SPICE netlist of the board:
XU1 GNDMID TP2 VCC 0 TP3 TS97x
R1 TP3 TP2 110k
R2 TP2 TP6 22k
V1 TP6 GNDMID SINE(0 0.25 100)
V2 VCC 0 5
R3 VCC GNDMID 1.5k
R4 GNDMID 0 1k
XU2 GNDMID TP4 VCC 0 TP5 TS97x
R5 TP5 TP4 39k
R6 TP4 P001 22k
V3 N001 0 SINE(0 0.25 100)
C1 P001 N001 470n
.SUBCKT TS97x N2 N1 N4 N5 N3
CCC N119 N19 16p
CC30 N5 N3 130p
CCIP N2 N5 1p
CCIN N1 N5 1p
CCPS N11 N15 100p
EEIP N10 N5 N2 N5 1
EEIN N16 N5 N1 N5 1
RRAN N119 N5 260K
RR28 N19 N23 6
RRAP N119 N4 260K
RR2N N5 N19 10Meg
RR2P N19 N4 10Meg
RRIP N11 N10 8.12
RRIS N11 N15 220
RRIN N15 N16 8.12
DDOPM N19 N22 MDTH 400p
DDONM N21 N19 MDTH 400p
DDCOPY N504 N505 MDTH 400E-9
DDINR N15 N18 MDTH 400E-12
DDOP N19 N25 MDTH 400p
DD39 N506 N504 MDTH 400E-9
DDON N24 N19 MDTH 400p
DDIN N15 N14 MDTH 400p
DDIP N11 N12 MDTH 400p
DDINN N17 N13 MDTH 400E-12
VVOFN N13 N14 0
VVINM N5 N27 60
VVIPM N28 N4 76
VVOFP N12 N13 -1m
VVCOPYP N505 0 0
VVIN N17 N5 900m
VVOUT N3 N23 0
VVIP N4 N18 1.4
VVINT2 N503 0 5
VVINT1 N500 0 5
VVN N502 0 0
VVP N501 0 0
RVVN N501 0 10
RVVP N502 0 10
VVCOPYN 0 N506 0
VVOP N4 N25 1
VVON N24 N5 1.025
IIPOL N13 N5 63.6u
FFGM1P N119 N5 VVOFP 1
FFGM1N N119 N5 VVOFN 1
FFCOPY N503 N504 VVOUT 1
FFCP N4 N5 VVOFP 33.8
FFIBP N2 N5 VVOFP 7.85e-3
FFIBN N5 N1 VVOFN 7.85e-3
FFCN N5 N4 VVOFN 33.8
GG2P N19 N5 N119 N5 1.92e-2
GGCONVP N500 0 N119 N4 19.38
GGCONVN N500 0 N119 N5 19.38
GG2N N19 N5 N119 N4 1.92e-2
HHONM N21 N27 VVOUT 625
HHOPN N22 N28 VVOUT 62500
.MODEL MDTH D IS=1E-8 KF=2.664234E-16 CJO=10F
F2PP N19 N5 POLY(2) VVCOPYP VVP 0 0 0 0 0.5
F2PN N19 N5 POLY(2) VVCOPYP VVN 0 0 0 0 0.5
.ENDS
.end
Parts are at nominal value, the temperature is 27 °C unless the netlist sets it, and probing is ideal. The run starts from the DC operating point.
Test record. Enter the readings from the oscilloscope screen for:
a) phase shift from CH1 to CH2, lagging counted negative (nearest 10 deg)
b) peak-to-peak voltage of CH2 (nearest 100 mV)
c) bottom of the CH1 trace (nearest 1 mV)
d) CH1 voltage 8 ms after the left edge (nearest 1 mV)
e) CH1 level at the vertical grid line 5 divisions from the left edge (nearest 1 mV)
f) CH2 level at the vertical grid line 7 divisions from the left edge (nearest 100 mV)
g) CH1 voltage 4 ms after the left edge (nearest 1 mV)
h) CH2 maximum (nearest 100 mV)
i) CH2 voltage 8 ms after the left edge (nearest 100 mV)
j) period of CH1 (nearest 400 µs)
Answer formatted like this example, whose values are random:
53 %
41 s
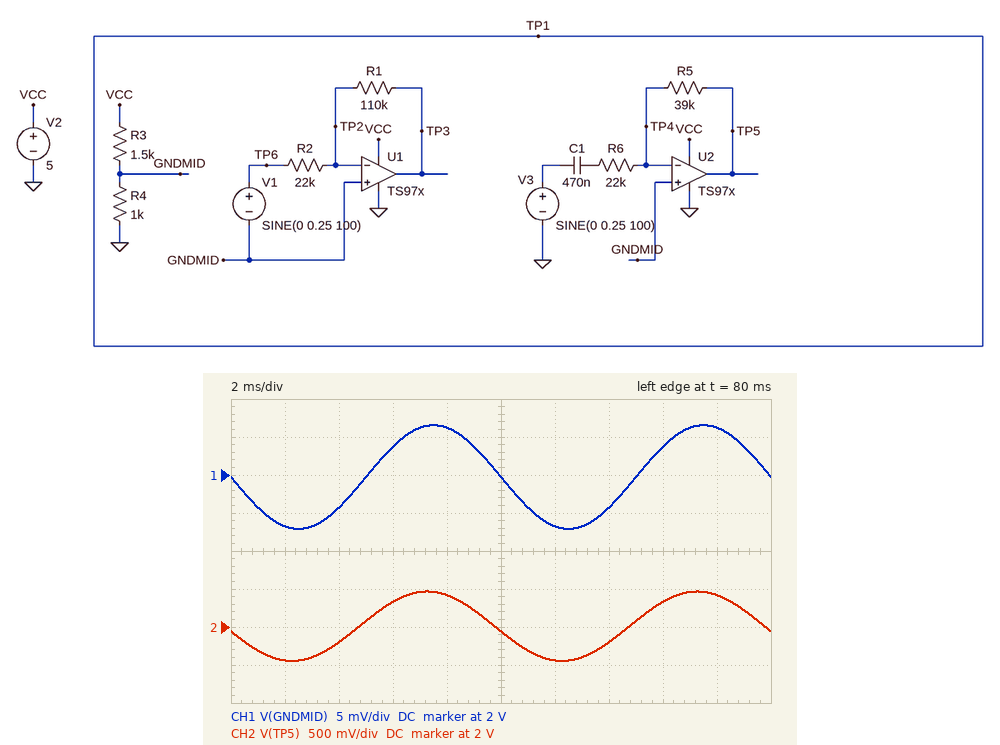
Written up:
10 deg
900 mV
1.993 V
2.006 V
2.000 V
1.8 V
1.996 V
2.5 V
2.4 V
10.0 ms
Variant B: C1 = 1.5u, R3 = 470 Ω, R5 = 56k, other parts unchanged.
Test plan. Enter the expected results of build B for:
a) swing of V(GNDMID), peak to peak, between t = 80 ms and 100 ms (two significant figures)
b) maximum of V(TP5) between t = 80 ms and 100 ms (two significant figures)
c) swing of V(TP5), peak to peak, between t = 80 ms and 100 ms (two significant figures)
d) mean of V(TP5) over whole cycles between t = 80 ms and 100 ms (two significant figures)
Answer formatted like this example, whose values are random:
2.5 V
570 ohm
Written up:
7.3 mV
4.1 V
1.3 V
3.4 V
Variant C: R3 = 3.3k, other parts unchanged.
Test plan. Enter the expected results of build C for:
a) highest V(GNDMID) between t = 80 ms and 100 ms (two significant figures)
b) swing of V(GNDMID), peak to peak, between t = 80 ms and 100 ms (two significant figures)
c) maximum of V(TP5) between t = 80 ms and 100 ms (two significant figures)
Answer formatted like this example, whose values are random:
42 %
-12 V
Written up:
1.2 V
17 mV
1.6 V
